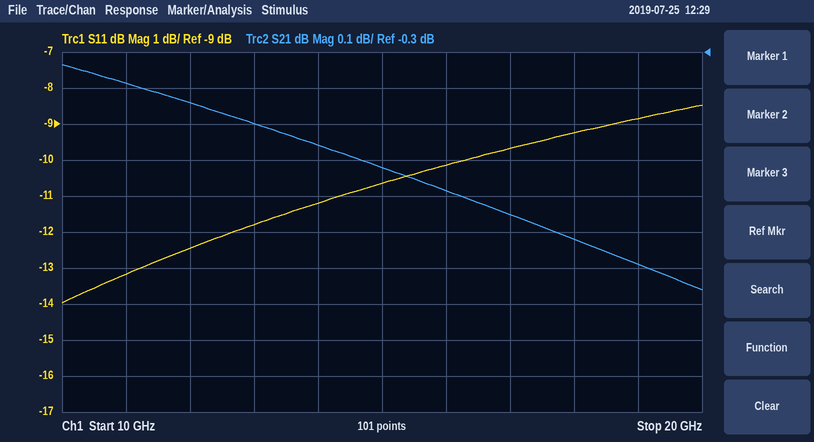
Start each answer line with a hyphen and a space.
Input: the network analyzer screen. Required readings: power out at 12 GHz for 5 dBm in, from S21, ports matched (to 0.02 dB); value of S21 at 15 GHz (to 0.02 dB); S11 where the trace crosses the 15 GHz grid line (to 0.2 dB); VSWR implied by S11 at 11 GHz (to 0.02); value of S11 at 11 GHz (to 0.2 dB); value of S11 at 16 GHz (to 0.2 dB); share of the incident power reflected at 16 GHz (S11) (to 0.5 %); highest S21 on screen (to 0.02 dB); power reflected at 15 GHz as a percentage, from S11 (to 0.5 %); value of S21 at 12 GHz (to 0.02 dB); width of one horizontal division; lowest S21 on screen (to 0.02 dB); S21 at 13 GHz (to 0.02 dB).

- 4.56 dBm
- -0.62 dB
- -10.6 dB
- 1.56
- -13.2 dB
- -10.2 dB
- 9.5 %
- -0.34 dB
- 8.5 %
- -0.44 dB
- 1 GHz
- -0.96 dB
- -0.50 dB
